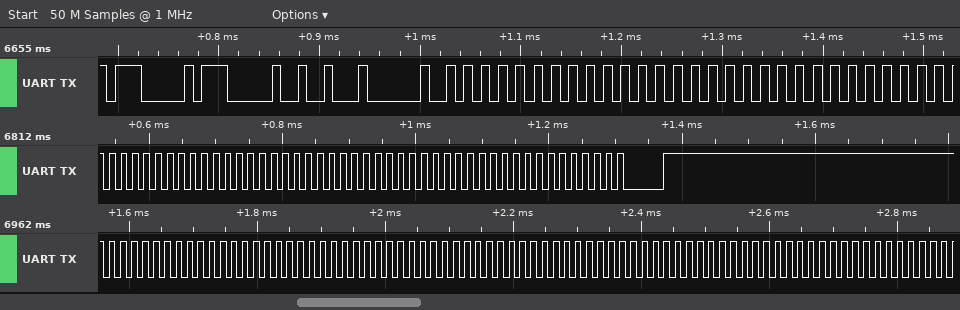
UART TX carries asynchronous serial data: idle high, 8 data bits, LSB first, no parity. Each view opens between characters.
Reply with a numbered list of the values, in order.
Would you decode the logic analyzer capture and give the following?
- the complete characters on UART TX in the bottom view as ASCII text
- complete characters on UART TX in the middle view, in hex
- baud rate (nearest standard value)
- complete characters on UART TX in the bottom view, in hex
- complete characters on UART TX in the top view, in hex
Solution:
1. "UUUUUUUUUUUUUUU"
2. 55, 55, 55, 55, 55, 55, 55, 55, 55, C0
3. 115200 baud
4. 55, 55, 55, 55, 55, 55, 55, 55, 55, 55, 55, 55, 55, 55, 55
5. 07, 07, 12, 20, 55, 55, 55, 55, 55
